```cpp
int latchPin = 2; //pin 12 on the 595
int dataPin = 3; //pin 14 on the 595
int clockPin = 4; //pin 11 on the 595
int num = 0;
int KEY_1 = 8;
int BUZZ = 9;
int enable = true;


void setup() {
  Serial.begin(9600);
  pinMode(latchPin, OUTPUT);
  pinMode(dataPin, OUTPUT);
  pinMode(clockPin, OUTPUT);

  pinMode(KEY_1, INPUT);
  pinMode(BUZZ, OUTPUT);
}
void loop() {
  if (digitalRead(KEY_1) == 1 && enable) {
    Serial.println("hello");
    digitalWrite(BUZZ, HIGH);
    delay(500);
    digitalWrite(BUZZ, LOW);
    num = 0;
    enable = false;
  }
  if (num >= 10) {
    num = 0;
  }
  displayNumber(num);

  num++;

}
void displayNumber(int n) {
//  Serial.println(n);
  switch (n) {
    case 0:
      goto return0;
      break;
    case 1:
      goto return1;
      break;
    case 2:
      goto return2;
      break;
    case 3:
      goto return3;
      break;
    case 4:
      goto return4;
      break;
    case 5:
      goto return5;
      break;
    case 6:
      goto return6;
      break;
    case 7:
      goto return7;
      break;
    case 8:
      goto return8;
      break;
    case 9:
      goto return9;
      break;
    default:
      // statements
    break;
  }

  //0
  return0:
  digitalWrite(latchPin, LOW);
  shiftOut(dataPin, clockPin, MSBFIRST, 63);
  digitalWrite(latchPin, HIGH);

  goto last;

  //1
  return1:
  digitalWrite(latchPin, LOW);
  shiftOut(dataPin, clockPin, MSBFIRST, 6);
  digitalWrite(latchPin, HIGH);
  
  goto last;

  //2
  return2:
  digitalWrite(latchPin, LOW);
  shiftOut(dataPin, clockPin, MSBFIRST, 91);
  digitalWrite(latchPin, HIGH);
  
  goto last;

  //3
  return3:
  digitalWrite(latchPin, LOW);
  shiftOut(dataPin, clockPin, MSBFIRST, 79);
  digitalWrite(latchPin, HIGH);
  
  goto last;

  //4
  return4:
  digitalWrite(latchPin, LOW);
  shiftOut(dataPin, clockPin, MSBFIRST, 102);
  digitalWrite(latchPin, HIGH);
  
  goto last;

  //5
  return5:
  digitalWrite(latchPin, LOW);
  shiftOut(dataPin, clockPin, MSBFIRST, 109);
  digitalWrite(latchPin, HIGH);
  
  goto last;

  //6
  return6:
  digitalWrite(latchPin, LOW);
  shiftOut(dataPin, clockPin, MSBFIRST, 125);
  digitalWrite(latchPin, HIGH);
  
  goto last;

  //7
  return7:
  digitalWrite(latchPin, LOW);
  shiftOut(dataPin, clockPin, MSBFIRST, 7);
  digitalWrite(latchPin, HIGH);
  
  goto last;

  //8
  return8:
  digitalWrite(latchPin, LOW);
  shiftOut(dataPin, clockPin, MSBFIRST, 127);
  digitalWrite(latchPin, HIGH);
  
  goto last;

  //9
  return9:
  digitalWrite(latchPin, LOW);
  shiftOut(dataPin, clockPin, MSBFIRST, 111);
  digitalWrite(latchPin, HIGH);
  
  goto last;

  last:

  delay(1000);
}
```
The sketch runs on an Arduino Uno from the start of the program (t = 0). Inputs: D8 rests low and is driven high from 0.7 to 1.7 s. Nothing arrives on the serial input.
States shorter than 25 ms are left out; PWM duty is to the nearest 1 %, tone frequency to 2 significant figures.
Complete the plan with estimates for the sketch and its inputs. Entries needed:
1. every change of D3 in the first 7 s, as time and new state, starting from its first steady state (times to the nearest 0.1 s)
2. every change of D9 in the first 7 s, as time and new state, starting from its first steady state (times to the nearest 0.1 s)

0 s high; 2.5 s low; 3.5 s high; 5.5 s low; 6.5 s high
0 s low; 1 s high; 1.5 s low
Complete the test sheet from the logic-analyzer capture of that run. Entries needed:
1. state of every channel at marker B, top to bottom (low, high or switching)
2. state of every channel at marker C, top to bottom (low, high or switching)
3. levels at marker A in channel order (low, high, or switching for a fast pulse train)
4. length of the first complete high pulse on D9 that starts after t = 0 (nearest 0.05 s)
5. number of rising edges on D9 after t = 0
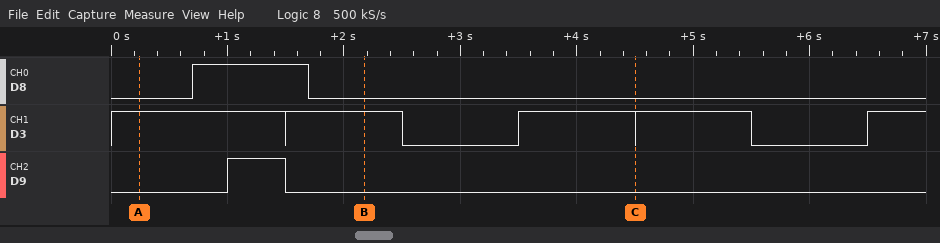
D8 low, D3 high, D9 low
D8 low, D3 high, D9 low
D8 low, D3 high, D9 low
0.50 s
1
